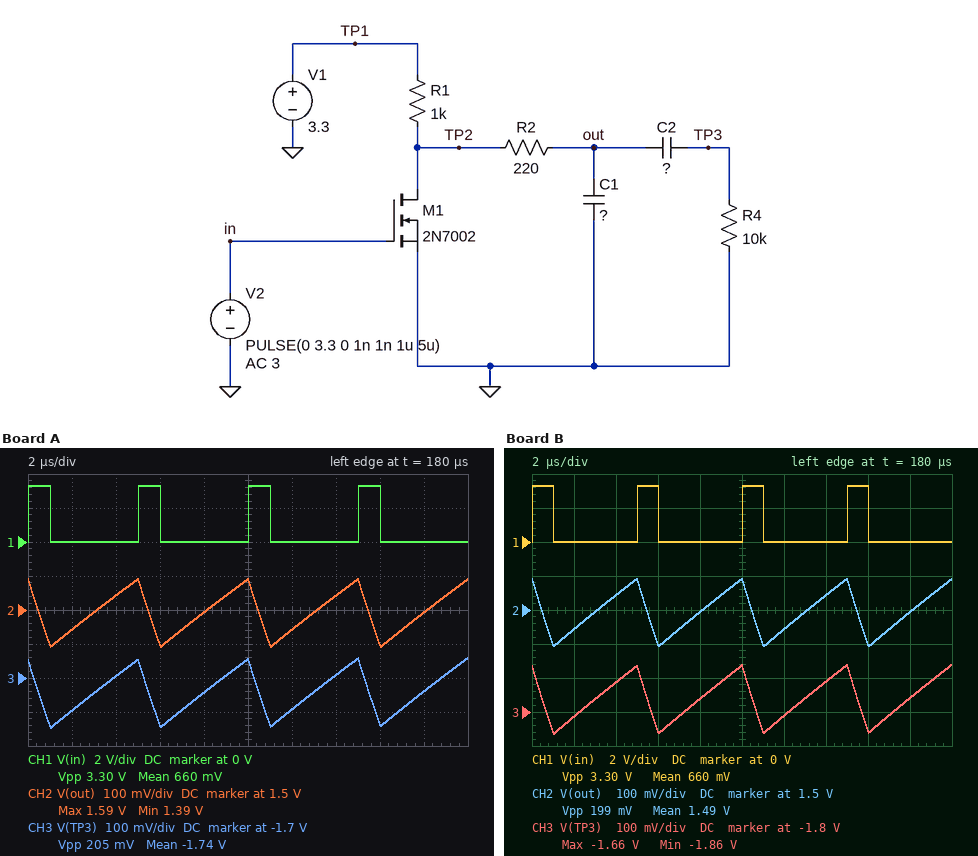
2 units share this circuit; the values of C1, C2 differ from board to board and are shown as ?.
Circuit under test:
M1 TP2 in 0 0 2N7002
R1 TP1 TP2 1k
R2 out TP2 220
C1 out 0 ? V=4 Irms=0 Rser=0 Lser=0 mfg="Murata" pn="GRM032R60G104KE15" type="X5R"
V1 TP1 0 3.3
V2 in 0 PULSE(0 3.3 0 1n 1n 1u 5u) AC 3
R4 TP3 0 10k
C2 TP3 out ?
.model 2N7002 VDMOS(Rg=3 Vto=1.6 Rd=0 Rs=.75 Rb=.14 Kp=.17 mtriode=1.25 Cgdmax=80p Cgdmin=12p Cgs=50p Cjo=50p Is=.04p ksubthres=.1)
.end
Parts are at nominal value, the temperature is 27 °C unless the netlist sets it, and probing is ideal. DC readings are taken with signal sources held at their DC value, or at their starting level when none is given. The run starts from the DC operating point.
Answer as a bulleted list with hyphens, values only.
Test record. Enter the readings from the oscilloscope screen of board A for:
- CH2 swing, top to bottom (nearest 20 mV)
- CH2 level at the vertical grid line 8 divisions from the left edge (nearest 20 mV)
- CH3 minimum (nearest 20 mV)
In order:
- 200 mV
- 1.40 V
- -1.84 V
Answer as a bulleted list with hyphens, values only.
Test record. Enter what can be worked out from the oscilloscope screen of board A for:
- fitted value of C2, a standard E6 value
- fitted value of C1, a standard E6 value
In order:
- 470 nF
- 33 nF
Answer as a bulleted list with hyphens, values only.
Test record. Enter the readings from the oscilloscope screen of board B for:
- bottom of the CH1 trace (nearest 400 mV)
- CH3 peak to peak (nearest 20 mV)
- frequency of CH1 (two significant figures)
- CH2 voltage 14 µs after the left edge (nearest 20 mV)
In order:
- 0 V
- 200 mV
- 200 kHz
- 1.54 V
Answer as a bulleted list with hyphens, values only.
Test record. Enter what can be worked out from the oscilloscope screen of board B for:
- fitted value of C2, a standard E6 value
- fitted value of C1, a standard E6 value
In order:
- 680 nF
- 33 nF
